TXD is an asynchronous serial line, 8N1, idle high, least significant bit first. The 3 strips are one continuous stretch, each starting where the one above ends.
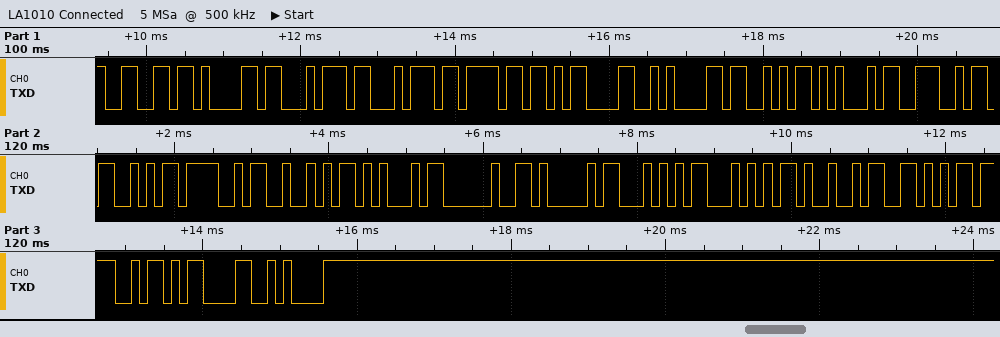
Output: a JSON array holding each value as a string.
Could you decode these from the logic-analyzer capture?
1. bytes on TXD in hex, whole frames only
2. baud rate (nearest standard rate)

["66 61 74 74 6F 0D 0A 53 45 4E 53 4F 52 45 20 41 54 54 49 56 4F 0D 0A", "9600 baud"]
